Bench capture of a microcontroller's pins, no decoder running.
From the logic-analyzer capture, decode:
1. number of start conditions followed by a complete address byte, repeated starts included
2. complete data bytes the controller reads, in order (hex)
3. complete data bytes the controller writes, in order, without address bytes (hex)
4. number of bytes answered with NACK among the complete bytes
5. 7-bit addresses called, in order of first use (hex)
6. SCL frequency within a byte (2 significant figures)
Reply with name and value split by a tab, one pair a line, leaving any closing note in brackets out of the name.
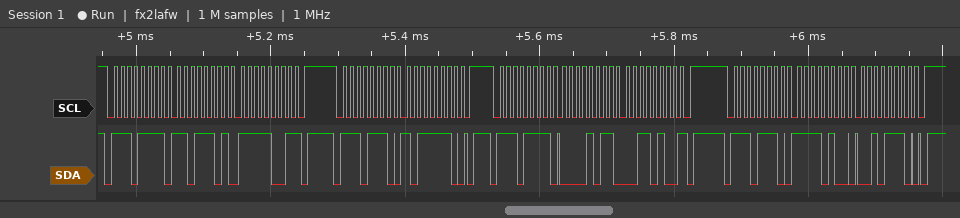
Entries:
number of start conditions followed by a complete address byte, repeated starts included	4
complete data bytes the controller reads, in order	DD F9 0B 34
complete data bytes the controller writes, in order, without address bytes	BE F4 2E
number of bytes answered with NACK among the complete bytes	2
7-bit addresses called, in order of first use	0x77
SCL frequency within a byte	100 kHz
